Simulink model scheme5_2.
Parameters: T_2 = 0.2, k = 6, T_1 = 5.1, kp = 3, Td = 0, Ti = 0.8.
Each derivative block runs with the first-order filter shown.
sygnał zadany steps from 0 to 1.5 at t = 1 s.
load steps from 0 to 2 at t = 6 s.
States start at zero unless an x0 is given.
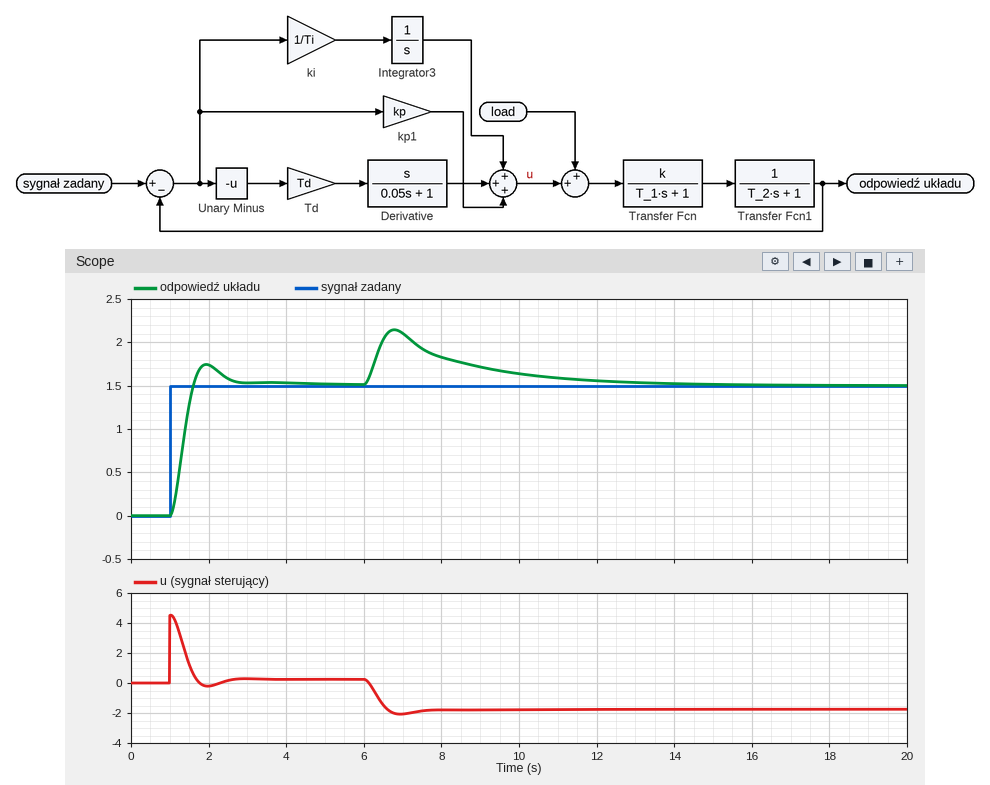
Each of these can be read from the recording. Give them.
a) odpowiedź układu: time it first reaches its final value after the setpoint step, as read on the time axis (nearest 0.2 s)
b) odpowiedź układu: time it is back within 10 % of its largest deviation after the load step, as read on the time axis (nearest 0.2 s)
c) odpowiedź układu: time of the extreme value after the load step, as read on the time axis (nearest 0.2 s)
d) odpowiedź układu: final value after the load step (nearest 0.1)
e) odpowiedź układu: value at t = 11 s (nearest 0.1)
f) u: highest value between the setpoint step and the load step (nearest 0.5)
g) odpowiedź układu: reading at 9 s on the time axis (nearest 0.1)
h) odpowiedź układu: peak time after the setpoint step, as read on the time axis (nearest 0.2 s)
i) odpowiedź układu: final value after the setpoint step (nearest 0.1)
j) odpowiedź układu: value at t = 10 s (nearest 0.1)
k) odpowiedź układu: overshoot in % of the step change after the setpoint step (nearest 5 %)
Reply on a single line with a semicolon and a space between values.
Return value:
1.6 s; 11.8 s; 6.8 s; 1.5; 1.6; 4.5; 1.7; 2.0 s; 1.5; 1.6; 15 %
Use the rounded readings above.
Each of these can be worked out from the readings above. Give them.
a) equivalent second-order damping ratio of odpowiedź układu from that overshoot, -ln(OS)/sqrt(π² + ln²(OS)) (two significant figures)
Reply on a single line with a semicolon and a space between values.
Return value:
0.52
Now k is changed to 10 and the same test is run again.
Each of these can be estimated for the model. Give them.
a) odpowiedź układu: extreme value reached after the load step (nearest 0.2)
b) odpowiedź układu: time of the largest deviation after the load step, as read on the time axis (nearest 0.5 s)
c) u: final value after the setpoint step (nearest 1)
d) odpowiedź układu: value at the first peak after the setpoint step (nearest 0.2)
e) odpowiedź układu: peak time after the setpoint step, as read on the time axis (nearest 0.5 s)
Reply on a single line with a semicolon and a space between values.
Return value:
2.2; 6.5 s; 0; 1.8; 1.5 s
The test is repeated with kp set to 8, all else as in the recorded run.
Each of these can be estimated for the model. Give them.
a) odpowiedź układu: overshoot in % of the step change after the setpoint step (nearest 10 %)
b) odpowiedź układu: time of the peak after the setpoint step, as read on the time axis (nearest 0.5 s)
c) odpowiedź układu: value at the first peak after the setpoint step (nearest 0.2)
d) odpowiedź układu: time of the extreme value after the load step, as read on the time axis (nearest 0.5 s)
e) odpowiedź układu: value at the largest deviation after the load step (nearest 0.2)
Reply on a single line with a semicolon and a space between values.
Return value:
30 %; 1.5 s; 2.0; 6.5 s; 1.8
